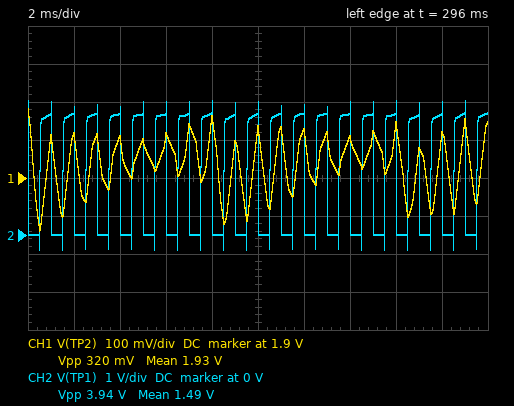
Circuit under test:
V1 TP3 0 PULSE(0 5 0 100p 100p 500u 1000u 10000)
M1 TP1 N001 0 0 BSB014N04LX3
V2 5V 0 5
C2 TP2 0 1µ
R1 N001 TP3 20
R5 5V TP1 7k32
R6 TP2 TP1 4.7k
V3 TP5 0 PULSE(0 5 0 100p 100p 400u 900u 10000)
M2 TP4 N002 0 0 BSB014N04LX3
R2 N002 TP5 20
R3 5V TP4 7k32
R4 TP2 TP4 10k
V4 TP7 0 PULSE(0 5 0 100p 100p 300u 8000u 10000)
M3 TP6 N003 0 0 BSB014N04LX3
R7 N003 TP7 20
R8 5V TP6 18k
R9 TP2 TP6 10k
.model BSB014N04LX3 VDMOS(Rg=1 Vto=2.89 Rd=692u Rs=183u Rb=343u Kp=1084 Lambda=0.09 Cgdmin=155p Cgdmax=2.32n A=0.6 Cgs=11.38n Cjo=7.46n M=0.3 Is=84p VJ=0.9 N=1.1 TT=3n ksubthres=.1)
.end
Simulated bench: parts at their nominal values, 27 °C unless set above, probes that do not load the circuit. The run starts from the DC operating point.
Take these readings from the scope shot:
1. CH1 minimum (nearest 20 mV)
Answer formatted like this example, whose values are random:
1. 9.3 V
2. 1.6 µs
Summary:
1. 1.76 V
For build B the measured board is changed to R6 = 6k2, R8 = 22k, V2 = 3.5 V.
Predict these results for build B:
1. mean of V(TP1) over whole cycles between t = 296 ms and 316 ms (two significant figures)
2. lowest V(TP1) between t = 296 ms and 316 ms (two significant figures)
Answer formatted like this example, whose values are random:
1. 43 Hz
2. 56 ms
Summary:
1. 1.1 V
2. -420 mV
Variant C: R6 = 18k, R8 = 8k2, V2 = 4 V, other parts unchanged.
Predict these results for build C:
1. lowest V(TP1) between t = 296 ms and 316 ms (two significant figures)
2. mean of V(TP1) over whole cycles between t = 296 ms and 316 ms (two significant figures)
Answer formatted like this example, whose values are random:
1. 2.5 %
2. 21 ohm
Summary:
1. -430 mV
2. 1.6 V
